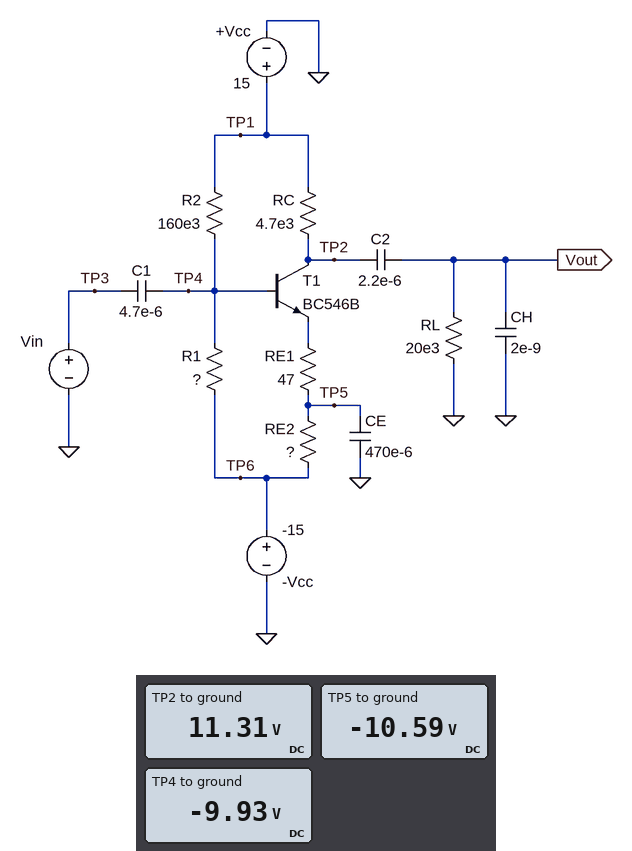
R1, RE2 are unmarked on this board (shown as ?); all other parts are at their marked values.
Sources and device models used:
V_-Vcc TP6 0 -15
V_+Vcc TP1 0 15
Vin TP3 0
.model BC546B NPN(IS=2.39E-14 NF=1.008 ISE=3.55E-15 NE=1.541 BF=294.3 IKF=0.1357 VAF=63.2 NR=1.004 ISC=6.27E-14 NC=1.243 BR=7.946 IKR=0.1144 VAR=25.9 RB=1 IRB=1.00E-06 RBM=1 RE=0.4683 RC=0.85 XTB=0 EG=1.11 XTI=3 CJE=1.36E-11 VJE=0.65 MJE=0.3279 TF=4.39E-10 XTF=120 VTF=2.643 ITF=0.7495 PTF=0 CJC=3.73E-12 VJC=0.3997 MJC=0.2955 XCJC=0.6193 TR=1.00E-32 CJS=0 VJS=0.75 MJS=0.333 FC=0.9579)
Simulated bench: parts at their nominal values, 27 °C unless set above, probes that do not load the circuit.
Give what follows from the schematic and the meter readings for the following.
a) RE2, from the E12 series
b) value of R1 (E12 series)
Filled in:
5.6 kΩ
33 kΩ
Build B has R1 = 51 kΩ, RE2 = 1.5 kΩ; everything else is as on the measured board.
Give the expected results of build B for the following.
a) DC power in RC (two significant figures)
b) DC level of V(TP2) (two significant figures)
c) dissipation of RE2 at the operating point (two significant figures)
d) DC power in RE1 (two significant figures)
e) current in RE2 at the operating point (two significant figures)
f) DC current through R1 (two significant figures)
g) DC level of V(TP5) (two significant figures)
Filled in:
72 mW
-3.4 V
23 mW
720 µW
3.9 mA
130 µA
-9.1 V
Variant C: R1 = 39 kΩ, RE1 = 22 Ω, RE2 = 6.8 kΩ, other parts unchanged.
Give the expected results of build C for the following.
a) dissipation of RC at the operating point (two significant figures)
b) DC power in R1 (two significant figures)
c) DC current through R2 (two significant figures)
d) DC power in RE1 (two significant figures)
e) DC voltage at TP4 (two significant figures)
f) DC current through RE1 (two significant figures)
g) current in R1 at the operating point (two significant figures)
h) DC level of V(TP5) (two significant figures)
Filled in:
2.7 mW
870 µW
150 µA
13 µW
-9.2 V
760 µA
150 µA
-9.8 V
